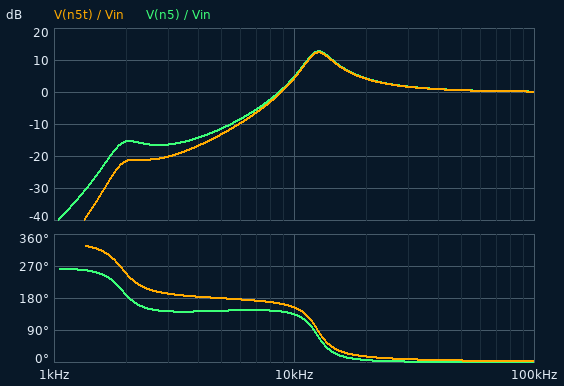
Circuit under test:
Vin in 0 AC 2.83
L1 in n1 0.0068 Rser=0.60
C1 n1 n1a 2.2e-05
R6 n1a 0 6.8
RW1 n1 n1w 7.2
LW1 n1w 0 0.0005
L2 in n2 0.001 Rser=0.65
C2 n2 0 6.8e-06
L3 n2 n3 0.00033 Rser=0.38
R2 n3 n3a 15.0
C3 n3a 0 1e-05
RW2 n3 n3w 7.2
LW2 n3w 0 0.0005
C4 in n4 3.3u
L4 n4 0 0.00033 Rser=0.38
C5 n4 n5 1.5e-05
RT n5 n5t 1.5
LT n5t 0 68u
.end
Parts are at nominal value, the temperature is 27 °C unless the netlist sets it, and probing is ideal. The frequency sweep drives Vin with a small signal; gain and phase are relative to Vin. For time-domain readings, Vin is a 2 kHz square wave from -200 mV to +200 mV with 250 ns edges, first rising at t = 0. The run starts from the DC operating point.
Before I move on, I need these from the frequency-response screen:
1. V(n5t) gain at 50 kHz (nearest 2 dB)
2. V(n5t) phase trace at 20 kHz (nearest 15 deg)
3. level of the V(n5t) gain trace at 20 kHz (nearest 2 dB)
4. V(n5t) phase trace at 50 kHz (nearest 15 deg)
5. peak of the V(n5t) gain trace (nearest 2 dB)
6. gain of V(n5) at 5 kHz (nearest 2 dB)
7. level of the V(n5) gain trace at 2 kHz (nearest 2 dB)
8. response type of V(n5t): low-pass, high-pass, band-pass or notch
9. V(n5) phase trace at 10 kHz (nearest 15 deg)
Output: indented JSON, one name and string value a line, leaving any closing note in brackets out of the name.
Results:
{
  "V(n5t) gain at 50 kHz": "0 dB",
  "V(n5t) phase trace at 20 kHz": "15 deg",
  "level of the V(n5t) gain trace at 20 kHz": "4 dB",
  "V(n5t) phase trace at 50 kHz": "0 deg",
  "peak of the V(n5t) gain trace": "12 dB",
  "gain of V(n5) at 5 kHz": "-12 dB",
  "level of the V(n5) gain trace at 2 kHz": "-16 dB",
  "response type of V(n5t): low-pass, high-pass, band-pass or notch": "high-pass",
  "V(n5) phase trace at 10 kHz": "135 deg"
}
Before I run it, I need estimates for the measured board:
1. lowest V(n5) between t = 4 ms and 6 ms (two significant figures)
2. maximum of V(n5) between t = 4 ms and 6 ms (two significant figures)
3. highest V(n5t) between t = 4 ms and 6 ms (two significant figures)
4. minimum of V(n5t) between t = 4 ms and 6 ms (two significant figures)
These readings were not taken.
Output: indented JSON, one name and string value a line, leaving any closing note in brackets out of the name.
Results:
{
  "lowest V(n5) between t = 4 ms and 6 ms": "-360 mV",
  "maximum of V(n5) between t = 4 ms and 6 ms": "360 mV",
  "highest V(n5t) between t = 4 ms and 6 ms": "360 mV",
  "minimum of V(n5t) between t = 4 ms and 6 ms": "-360 mV"
}
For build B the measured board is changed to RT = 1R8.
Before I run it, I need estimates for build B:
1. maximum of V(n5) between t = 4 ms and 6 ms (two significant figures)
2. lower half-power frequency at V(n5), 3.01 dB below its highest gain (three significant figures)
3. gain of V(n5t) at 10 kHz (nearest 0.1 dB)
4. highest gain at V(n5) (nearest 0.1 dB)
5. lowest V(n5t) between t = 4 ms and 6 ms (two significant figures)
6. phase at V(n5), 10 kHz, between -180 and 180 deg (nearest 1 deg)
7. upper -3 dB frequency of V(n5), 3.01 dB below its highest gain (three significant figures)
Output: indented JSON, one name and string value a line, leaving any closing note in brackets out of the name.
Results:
{
  "maximum of V(n5) between t = 4 ms and 6 ms": "370 mV",
  "lower half-power frequency at V(n5), 3.01 dB below its highest gain": "11.1 kHz",
  "gain of V(n5t) at 10 kHz": "3.8 dB",
  "highest gain at V(n5)": "11.3 dB",
  "lowest V(n5t) between t = 4 ms and 6 ms": "-370 mV",
  "phase at V(n5), 10 kHz, between -180 and 180 deg": "127 deg",
  "upper -3 dB frequency of V(n5), 3.01 dB below its highest gain": "15.2 kHz"
}
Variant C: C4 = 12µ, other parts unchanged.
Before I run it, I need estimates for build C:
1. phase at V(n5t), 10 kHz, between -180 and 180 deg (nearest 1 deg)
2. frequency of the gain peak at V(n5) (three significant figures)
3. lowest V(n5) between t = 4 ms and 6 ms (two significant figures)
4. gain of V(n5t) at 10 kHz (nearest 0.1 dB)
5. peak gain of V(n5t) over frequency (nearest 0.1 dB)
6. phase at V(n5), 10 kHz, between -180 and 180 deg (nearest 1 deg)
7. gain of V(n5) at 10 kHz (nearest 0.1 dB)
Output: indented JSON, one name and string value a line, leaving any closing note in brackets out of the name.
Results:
{
  "phase at V(n5t), 10 kHz, between -180 and 180 deg": "40 deg",
  "frequency of the gain peak at V(n5)": "7.95 kHz",
  "lowest V(n5) between t = 4 ms and 6 ms": "-430 mV",
  "gain of V(n5t) at 10 kHz": "5.8 dB",
  "peak gain of V(n5t) over frequency": "7.9 dB",
  "phase at V(n5), 10 kHz, between -180 and 180 deg": "21 deg",
  "gain of V(n5) at 10 kHz": "6.3 dB"
}
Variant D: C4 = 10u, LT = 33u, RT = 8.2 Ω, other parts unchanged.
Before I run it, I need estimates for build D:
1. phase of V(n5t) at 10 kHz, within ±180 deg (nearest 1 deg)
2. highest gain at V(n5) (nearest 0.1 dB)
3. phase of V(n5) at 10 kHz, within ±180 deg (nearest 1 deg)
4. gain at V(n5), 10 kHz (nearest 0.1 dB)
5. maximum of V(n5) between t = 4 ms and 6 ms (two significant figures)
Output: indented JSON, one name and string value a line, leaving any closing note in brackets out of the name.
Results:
{
  "phase of V(n5t) at 10 kHz, within ±180 deg": "95 deg",
  "highest gain at V(n5)": "2.4 dB",
  "phase of V(n5) at 10 kHz, within ±180 deg": "19 deg",
  "gain at V(n5), 10 kHz": "0.9 dB",
  "maximum of V(n5) between t = 4 ms and 6 ms": "400 mV"
}
